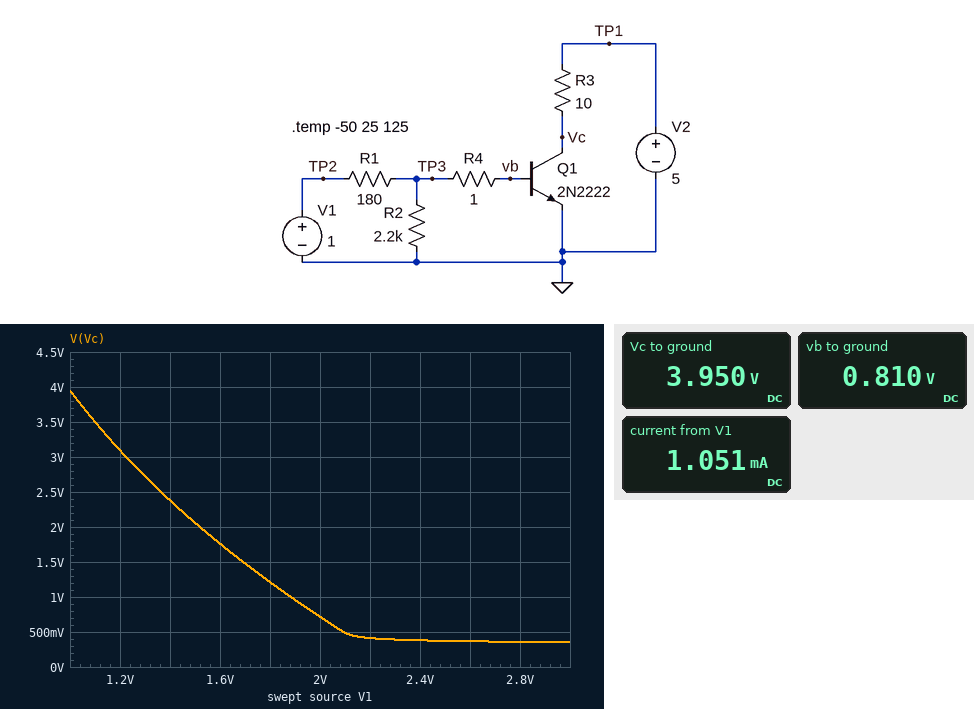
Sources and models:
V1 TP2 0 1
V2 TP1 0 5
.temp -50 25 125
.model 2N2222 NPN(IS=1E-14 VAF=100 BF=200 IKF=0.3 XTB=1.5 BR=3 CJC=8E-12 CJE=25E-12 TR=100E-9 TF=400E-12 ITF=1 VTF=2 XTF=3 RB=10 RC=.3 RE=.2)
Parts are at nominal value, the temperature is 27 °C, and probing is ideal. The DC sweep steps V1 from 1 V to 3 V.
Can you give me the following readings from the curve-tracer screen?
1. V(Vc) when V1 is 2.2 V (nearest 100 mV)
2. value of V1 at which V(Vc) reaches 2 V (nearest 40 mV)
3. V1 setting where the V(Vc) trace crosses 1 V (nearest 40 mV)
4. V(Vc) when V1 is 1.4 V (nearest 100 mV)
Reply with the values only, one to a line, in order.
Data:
400 mV
1.52 V
1.88 V
2.4 V
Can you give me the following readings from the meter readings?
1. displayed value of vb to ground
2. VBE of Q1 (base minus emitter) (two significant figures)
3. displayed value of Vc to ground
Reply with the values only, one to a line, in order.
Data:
0.810 V
810 mV
3.950 V
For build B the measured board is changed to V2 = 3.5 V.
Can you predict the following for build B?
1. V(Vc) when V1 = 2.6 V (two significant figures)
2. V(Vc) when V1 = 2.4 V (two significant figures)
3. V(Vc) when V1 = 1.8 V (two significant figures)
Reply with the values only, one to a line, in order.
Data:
260 mV
270 mV
300 mV
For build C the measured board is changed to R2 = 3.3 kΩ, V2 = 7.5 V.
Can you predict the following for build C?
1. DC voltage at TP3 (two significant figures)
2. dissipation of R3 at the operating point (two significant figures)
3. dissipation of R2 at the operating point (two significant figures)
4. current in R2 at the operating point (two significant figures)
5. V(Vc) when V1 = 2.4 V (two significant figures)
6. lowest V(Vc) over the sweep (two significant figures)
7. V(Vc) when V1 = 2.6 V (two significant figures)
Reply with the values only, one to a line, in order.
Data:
820 mV
140 mW
200 µW
250 µA
2.2 V
1.0 V
1.8 V
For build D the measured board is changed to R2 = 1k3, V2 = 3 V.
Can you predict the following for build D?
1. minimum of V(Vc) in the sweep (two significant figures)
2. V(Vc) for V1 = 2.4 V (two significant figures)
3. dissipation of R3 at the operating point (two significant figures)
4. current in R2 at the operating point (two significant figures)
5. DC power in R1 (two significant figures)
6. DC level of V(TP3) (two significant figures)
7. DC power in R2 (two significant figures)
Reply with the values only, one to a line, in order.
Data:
230 mV
240 mV
67 mW
610 µA
230 µW
800 mV
490 µW
